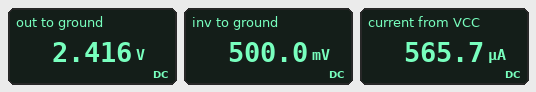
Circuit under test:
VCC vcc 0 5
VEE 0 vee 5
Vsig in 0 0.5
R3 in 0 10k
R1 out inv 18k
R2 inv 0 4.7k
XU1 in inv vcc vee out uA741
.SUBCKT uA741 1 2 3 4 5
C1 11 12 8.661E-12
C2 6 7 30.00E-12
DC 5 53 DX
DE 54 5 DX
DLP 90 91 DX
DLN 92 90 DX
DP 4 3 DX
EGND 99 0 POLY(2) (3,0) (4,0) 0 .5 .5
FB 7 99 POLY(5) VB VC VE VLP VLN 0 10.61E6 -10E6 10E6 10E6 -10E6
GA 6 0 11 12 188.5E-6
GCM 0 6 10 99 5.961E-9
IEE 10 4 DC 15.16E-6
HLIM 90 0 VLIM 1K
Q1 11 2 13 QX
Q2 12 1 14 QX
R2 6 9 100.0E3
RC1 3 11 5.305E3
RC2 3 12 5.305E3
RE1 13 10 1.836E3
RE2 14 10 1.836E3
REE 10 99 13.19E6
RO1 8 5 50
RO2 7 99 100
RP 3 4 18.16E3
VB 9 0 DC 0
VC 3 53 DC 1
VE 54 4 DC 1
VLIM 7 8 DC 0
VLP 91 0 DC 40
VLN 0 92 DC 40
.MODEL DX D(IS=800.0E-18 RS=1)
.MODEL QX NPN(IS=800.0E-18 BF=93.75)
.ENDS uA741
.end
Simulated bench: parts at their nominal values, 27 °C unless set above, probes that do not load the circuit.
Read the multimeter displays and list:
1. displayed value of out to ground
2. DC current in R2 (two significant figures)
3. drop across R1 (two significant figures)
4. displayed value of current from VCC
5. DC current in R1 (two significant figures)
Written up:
2.416 V
110 µA
1.9 V
565.7 µA
110 µA
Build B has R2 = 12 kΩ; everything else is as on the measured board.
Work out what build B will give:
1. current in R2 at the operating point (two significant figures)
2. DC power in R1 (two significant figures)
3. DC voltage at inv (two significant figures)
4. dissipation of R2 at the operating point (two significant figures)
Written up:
42 µA
31 µW
500 mV
21 µW
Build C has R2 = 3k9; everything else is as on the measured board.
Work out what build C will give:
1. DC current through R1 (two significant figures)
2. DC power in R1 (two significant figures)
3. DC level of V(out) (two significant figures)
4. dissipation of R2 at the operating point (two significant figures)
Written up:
130 µA
300 µW
2.8 V
64 µW
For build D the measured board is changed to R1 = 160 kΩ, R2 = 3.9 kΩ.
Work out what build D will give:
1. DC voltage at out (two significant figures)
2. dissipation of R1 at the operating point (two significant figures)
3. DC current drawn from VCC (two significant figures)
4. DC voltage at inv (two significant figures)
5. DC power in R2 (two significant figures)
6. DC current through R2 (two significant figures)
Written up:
4.6 V
130 µW
550 µA
110 mV
3.1 µW
28 µA
